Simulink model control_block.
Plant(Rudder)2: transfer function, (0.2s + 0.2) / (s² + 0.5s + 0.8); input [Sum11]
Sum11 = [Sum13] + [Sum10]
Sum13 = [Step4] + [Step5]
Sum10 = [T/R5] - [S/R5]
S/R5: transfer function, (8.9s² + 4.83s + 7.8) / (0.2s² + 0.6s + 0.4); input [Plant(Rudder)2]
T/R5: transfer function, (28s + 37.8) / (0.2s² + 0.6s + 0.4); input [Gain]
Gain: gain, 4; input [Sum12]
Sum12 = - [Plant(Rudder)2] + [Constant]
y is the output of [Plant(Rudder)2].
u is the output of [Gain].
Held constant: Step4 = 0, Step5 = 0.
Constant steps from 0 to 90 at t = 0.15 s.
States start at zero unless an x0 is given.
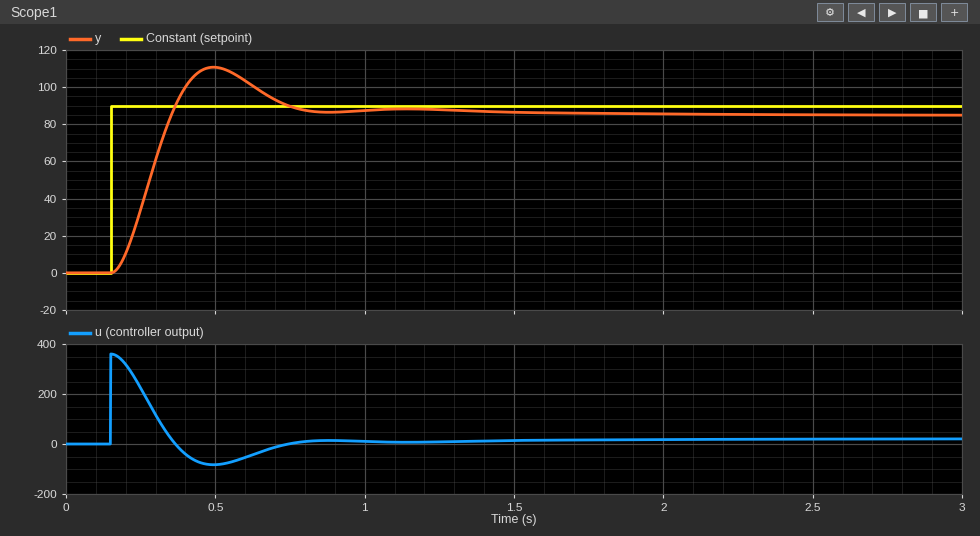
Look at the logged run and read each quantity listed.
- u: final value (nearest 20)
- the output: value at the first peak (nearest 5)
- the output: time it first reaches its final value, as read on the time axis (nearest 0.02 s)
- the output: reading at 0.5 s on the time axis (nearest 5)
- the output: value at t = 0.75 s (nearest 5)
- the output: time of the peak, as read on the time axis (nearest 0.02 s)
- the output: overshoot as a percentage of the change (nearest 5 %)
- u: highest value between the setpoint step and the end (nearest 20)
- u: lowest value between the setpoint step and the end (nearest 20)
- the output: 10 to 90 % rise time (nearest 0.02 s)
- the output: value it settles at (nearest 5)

20
110
0.36 s
110
90
0.50 s
30 %
360
-80
0.14 s
85
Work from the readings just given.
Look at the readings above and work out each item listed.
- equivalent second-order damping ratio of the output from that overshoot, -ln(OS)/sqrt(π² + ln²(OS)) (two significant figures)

0.36
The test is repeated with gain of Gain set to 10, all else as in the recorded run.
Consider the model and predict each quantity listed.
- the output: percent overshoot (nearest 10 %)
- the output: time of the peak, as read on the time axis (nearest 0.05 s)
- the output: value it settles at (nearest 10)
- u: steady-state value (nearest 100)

40 %
0.35 s
90
0
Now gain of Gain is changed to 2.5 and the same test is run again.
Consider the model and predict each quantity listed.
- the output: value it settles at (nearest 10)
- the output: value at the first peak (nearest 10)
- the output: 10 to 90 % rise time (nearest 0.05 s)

80
100
0.20 s
